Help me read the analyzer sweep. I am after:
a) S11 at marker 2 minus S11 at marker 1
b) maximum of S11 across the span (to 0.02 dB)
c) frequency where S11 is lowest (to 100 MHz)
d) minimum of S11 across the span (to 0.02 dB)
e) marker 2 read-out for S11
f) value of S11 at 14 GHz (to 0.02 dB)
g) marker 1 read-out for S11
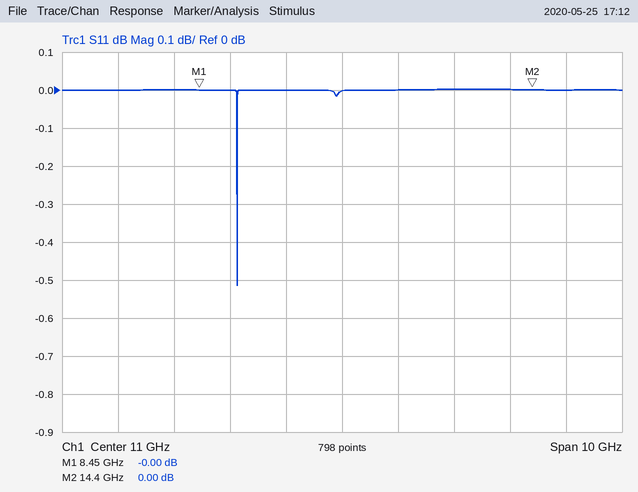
0.00 dB
0.00 dB
9.1 GHz
-0.52 dB
0.00 dB
0.00 dB
-0.00 dB
